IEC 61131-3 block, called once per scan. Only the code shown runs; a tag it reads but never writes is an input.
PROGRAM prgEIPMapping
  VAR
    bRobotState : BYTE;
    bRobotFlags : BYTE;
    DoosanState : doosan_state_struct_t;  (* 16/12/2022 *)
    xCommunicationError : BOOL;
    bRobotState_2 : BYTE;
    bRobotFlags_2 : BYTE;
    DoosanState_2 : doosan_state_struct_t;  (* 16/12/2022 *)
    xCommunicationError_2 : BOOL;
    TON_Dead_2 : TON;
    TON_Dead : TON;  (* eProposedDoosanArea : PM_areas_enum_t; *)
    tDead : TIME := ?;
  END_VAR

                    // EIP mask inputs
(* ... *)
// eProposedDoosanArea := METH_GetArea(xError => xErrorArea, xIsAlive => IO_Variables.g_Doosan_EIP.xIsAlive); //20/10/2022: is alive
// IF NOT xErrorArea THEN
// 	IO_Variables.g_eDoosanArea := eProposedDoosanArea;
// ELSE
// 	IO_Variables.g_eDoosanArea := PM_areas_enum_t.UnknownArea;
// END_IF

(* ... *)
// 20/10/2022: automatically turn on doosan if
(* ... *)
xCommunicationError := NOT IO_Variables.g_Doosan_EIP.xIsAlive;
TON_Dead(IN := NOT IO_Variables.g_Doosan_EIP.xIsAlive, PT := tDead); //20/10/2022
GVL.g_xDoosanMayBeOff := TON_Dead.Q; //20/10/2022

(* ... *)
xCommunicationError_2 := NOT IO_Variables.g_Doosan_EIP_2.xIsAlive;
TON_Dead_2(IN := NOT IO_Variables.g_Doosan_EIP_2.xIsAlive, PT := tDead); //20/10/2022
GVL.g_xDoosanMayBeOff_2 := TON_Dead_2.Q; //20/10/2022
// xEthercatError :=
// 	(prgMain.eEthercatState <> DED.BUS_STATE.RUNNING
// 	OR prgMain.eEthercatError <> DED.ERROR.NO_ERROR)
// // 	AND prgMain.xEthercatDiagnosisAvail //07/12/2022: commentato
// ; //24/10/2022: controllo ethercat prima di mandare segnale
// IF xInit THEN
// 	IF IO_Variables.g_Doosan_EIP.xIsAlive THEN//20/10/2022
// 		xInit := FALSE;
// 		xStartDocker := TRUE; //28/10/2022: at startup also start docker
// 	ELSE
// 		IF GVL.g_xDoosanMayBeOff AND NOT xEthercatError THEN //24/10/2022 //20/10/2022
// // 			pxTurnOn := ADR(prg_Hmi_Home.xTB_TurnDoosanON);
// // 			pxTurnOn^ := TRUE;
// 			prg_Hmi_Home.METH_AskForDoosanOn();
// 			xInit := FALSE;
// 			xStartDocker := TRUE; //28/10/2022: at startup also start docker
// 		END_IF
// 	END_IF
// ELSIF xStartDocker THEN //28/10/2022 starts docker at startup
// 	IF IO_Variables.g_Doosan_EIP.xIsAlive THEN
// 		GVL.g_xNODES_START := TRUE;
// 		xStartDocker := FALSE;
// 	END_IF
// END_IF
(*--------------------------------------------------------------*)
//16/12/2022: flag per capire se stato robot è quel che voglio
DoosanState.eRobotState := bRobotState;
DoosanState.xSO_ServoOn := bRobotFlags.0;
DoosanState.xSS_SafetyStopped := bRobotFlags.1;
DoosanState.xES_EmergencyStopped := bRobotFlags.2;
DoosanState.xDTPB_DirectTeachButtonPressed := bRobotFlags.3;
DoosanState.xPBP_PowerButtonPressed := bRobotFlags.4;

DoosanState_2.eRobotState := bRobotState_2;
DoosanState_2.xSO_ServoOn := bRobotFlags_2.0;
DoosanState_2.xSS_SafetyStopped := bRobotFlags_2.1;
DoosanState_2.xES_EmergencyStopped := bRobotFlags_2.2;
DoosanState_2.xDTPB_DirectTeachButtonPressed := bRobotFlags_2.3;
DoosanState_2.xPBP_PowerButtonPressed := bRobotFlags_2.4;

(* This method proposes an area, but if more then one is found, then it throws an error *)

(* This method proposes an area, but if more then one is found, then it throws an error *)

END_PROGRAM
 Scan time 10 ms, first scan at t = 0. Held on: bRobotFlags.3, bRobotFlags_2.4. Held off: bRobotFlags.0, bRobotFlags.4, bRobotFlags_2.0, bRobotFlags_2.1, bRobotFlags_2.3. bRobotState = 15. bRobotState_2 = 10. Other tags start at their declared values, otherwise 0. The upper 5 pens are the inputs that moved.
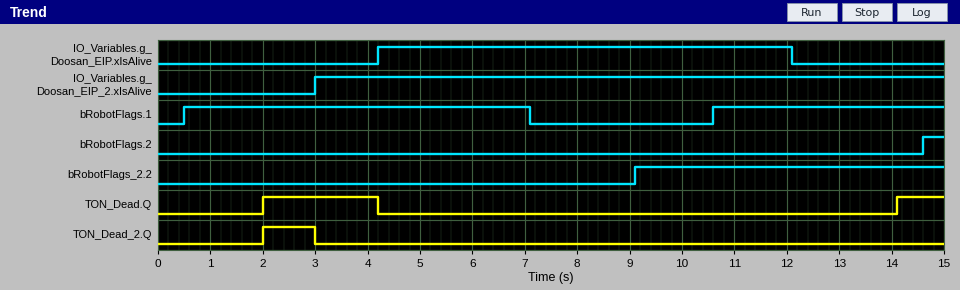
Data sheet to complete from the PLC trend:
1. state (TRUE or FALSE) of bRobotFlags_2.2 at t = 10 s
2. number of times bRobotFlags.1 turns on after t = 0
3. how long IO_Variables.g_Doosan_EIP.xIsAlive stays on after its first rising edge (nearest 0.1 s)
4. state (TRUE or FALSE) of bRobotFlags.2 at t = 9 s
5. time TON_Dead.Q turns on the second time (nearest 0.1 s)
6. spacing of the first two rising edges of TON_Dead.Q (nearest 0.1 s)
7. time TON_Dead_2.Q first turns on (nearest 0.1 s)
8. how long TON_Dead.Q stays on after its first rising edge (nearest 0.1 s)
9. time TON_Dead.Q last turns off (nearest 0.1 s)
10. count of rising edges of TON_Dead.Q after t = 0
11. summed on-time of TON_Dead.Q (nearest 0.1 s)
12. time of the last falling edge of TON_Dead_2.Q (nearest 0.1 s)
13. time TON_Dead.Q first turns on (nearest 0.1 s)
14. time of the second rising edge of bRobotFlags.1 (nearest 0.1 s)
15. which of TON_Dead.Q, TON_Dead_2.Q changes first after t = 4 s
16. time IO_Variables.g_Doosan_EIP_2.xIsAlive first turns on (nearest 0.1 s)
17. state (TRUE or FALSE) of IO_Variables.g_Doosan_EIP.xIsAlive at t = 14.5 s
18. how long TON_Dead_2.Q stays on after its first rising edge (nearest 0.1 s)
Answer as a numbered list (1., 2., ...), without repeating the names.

1. TRUE
2. 2
3. 7.9 s
4. FALSE
5. 14.1 s
6. 12.1 s
7. 2.0 s
8. 2.2 s
9. 4.2 s
10. 2
11. 3.1 s
12. 3.0 s
13. 2.0 s
14. 10.6 s
15. TON_Dead.Q
16. 3.0 s
17. FALSE
18. 1.0 s
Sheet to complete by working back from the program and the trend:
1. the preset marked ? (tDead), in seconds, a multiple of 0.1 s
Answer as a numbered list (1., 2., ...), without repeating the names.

1. 2.0 s
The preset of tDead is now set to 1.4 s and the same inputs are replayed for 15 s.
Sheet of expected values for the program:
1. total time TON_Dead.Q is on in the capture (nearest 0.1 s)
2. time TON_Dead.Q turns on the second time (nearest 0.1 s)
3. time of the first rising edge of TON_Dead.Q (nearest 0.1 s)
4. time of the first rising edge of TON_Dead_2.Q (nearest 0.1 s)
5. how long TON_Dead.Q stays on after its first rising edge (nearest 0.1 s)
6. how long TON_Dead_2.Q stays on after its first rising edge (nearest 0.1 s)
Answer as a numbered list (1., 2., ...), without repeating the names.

1. 4.3 s
2. 13.5 s
3. 1.4 s
4. 1.4 s
5. 2.8 s
6. 1.6 s
